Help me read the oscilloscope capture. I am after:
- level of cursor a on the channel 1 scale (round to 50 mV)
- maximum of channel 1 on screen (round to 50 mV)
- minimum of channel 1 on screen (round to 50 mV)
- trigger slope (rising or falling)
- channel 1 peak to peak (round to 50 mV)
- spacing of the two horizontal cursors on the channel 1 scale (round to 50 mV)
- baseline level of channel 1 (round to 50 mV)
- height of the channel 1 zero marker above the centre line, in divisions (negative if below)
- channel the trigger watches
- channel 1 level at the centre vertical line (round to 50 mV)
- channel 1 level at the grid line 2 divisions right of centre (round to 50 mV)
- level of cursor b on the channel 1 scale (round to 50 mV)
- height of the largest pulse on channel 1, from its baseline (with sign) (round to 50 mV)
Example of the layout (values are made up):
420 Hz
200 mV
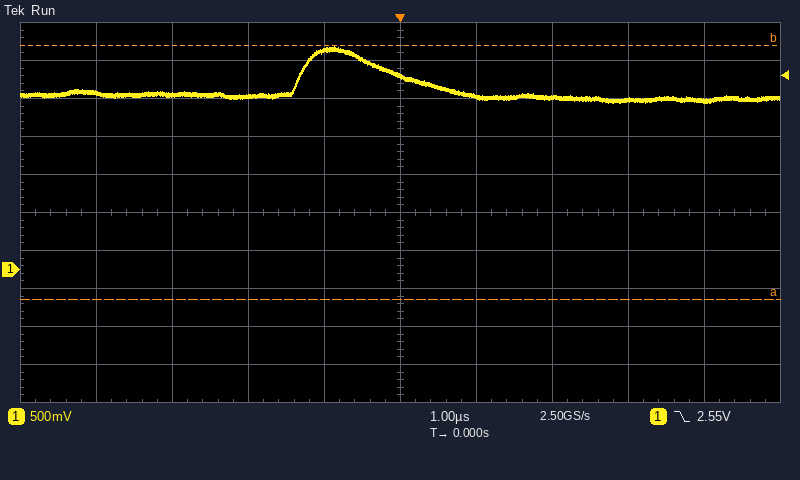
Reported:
-400 mV
2.95 V
2.20 V
falling
750 mV
3.35 V
2.30 V
-1.5 div
channel 1
2.55 V
2.25 V
2.95 V
+650 mV
